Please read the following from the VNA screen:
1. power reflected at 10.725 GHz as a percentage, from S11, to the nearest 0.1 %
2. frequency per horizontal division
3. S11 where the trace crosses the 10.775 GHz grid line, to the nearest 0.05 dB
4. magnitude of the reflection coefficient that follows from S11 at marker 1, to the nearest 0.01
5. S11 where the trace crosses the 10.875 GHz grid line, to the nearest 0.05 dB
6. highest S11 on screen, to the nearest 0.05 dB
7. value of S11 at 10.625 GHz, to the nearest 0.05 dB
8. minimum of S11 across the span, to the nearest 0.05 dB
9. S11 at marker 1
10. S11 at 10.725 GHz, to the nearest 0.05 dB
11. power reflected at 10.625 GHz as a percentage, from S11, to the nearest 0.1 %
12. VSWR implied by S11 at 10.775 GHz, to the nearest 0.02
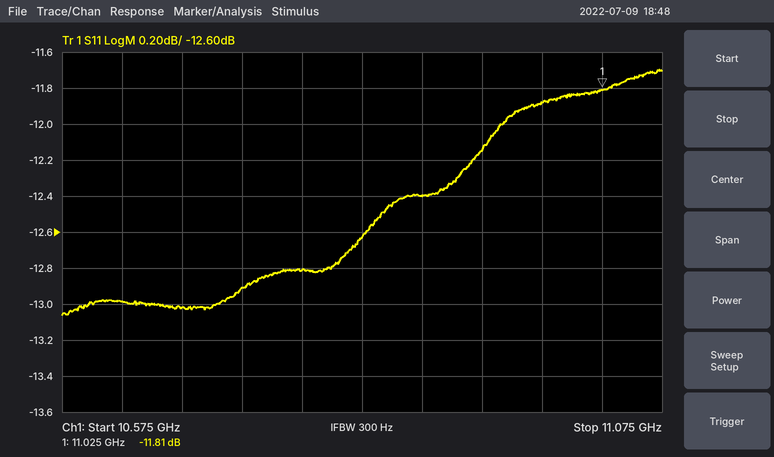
5.1 %
50 MHz
-12.80 dB
0.26
-12.40 dB
-11.70 dB
-13.00 dB
-13.05 dB
-11.81 dB
-12.90 dB
5.0 %
1.60
